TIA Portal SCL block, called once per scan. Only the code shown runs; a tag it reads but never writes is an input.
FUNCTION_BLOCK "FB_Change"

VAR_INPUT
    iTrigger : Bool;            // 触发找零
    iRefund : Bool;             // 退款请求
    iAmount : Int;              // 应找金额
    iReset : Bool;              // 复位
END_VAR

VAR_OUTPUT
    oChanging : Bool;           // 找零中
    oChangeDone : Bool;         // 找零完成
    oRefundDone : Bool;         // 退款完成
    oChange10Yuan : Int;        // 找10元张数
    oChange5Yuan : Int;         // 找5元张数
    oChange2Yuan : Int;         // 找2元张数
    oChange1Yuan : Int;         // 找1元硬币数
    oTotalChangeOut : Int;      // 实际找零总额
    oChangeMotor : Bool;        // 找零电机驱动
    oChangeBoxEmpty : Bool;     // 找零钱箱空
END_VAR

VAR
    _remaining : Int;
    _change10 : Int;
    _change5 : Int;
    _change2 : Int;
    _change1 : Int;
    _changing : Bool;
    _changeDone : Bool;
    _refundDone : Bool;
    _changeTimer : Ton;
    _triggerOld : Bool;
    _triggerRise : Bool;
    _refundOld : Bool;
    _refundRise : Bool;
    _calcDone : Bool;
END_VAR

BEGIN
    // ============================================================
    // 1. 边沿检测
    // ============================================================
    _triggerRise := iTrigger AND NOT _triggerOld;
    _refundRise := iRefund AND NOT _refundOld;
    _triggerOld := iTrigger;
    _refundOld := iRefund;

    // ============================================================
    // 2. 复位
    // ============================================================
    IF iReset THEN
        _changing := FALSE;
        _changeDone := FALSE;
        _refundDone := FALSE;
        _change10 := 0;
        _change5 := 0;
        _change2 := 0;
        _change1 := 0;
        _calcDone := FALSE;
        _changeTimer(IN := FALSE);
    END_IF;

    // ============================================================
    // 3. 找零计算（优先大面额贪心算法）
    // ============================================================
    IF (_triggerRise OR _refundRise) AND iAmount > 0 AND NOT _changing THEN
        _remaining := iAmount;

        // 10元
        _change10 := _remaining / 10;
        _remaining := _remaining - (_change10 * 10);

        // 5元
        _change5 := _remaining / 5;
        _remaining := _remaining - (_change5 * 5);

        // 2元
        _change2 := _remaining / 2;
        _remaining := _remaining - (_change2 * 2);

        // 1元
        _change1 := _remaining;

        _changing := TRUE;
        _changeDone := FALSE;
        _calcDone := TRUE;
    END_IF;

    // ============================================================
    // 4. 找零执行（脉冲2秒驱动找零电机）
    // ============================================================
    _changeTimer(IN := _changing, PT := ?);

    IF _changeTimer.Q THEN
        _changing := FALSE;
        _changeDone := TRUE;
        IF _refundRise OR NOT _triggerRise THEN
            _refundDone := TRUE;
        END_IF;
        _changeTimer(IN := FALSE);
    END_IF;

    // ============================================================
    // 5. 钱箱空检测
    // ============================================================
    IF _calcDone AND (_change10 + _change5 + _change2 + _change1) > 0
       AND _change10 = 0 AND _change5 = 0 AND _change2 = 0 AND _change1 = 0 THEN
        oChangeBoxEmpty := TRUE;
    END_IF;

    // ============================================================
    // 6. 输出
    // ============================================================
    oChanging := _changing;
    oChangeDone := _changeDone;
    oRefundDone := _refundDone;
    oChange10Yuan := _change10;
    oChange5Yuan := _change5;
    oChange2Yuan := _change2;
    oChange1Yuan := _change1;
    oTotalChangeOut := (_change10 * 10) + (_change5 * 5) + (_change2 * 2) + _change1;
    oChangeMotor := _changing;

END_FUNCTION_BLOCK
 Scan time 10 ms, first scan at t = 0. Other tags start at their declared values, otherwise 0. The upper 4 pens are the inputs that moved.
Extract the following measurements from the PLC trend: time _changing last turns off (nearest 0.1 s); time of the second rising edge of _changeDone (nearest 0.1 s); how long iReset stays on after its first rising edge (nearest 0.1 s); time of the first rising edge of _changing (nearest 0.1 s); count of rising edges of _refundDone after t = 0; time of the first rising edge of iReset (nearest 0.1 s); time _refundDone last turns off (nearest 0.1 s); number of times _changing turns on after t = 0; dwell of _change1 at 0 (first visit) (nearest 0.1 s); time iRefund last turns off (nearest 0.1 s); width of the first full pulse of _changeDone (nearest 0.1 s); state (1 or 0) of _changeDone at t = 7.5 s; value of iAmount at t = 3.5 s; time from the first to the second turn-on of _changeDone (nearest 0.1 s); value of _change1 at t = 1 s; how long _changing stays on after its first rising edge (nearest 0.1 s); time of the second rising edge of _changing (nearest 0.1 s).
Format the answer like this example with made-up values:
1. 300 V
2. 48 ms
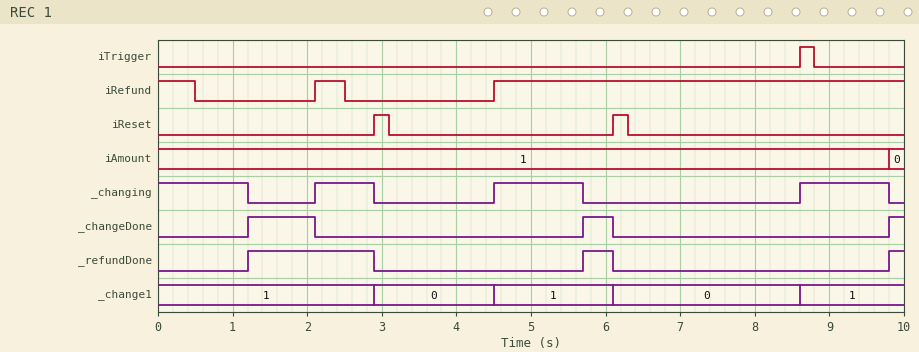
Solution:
1. 9.8 s
2. 5.7 s
3. 0.2 s
4. 2.1 s
5. 3
6. 2.9 s
7. 6.1 s
8. 3
9. 1.6 s
10. 2.5 s
11. 0.9 s
12. 0
13. 1
14. 4.5 s
15. 1
16. 0.8 s
17. 4.5 s
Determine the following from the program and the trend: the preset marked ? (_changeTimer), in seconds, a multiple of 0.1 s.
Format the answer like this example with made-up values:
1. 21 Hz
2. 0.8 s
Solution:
1. 1.2 s
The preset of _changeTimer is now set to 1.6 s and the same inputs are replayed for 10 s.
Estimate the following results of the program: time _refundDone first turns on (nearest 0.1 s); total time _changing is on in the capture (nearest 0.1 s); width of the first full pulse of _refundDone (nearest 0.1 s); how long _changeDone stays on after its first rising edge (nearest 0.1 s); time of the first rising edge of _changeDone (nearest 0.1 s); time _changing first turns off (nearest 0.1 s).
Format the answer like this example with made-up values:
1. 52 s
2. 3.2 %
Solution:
1. 1.6 s
2. 5.4 s
3. 1.3 s
4. 0.5 s
5. 1.6 s
6. 1.6 s
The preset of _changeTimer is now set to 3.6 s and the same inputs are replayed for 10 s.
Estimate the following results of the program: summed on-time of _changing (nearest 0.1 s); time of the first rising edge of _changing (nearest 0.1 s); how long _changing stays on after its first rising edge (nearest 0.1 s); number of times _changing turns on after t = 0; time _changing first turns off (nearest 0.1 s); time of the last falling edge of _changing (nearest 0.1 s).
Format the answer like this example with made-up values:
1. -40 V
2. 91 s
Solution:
1. 5.9 s
2. 4.5 s
3. 1.6 s
4. 2
5. 2.9 s
6. 6.1 s
